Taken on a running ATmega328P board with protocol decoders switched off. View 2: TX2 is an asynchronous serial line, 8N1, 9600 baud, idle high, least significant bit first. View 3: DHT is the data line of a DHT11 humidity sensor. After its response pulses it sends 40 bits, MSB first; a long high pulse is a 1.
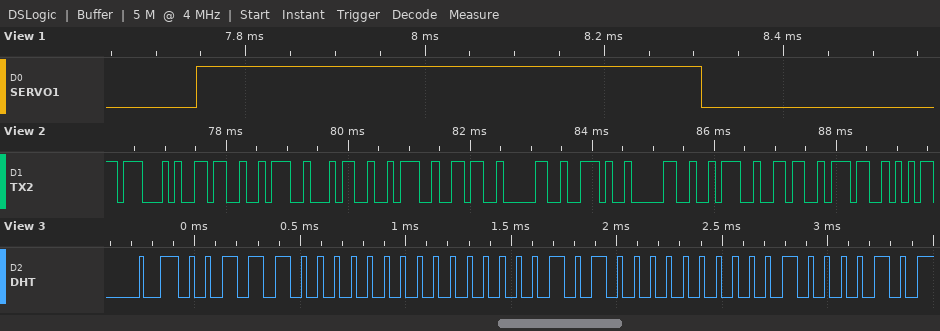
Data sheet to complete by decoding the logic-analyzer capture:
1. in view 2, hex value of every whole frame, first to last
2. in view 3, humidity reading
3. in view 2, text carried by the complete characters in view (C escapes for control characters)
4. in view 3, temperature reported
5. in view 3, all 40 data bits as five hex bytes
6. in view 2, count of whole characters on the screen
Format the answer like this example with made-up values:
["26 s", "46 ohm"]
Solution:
["0x47 0x36 0x3A 0x34 0x3A 0x36 0x30 0x2E 0x30 0x3A 0x36 0x37", "56 %", "\"G6:4:60.0:67\"", "10.0 °C", "38 00 0A 00 42", "12"]
